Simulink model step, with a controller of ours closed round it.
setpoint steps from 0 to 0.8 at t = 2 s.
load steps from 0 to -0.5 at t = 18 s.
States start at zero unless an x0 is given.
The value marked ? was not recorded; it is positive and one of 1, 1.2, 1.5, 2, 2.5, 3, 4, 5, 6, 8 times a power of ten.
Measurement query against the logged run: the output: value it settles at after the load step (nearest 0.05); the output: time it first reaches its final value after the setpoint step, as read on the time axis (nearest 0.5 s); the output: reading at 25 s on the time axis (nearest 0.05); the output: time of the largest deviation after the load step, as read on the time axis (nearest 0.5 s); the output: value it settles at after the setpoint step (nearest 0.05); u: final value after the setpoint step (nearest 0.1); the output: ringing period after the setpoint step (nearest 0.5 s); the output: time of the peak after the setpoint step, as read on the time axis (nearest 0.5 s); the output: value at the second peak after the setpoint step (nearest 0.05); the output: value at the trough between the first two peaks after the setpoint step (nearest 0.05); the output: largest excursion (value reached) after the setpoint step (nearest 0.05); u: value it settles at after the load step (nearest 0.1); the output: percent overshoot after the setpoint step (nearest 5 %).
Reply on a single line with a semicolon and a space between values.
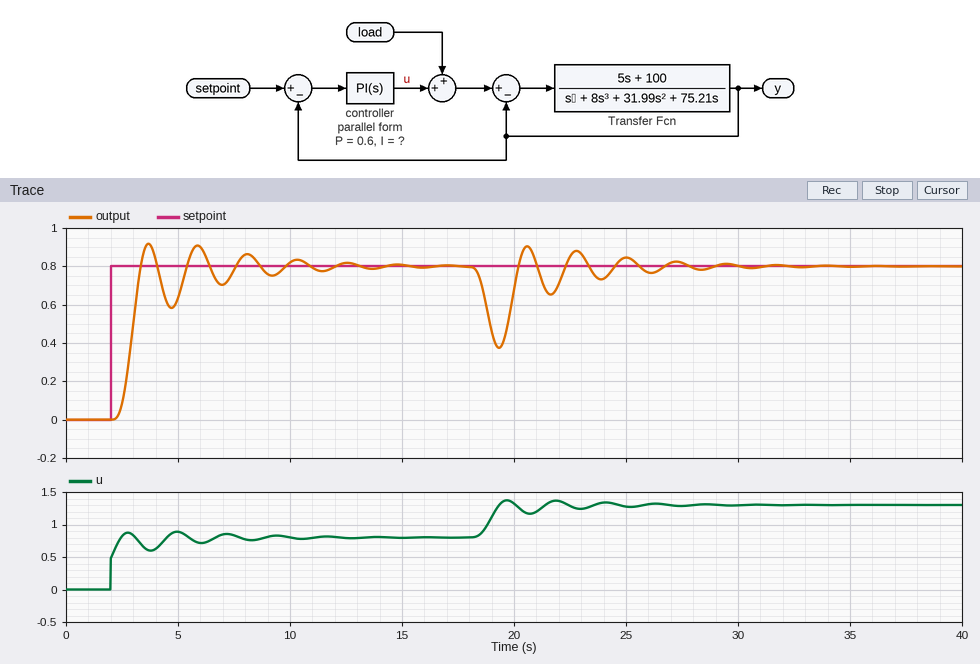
0.80; 3.5 s; 0.85; 19.5 s; 0.80; 0.8; 2.0 s; 3.5 s; 0.90; 0.60; 0.90; 1.3; 15 %
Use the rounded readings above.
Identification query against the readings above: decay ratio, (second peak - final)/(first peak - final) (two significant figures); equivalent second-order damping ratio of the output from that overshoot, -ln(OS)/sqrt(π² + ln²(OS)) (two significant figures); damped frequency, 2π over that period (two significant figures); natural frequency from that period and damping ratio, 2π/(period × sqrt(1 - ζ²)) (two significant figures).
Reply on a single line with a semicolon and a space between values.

1.0; 0.52; 3.1 rad/s; 3.7 rad/s
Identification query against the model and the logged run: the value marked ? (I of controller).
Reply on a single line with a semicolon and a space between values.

1
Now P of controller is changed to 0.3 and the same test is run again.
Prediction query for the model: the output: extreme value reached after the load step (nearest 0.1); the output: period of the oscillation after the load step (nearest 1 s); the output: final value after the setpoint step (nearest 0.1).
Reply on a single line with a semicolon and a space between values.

0.3; 3 s; 0.8
